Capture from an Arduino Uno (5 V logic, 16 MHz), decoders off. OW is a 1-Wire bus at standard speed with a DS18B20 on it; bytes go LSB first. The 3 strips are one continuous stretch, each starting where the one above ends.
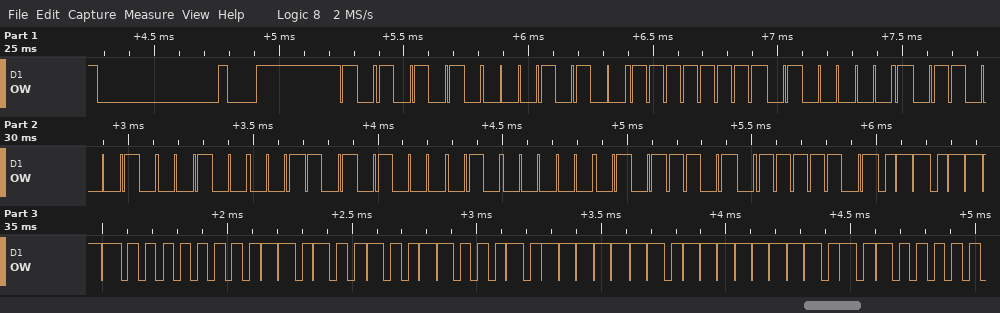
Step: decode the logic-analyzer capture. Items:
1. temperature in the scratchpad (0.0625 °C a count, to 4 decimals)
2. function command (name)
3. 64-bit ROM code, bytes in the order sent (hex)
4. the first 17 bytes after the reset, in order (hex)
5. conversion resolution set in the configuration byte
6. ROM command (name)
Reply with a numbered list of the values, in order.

1. 15.3750 °C
2. Read Scratchpad
3. 28 FF 82 46 84 15 02 BA
4. 55 28 FF 82 46 84 15 02 BA BE F6 00 4B 46 7F FF 0A
5. 12 bits
6. Match ROM
